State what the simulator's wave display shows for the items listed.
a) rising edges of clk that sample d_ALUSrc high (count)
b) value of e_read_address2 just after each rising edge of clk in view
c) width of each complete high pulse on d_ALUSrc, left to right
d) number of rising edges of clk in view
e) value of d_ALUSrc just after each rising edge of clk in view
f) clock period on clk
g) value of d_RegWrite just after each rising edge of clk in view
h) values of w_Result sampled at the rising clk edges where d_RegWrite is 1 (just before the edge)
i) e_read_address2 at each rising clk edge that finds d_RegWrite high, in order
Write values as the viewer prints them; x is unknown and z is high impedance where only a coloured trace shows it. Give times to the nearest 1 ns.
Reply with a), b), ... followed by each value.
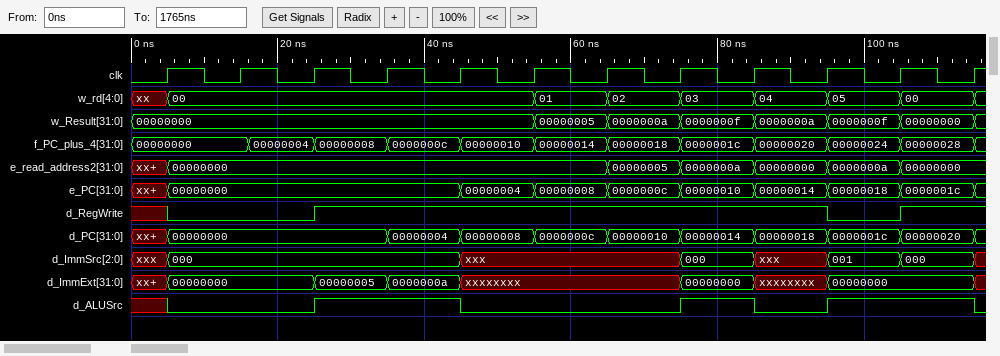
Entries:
a) 5
b) 00000000, 00000000, 00000000, 00000000, 00000000, 00000000, 00000005, 0000000a, 00000000, 0000000a, 00000000, 00000000
c) 20 ns, 10 ns, 20 ns
d) 12
e) 0 0 1 1 0 0 0 1 0 1 1 0
f) 10 ns
g) 0 0 1 1 1 1 1 1 1 0 1 1
h) 00000000, 00000000, 00000000, 00000005, 0000000a, 0000000f, 0000000a, 00000000
i) 00000000, 00000000, 00000000, 00000000, 00000005, 0000000a, 00000000, 00000000
